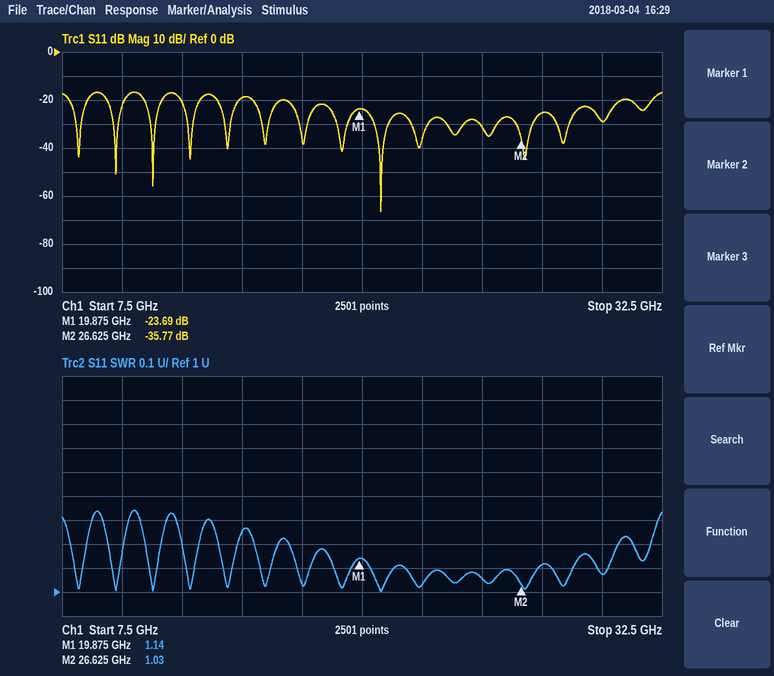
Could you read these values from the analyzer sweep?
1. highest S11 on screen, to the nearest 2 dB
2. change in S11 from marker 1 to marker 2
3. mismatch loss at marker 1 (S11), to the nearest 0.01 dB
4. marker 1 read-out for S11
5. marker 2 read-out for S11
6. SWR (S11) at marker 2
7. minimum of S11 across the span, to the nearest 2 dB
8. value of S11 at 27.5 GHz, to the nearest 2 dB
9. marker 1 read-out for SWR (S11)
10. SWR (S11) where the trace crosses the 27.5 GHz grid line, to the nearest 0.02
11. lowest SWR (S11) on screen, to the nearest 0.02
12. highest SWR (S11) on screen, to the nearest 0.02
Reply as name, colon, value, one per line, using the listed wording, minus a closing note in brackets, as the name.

highest S11 on screen, to the nearest 2 dB: -16 dB
change in S11 from marker 1 to marker 2: -12.08 dB
mismatch loss at marker 1 (S11), to the nearest 0.01 dB: 0.02 dB
marker 1 read-out for S11: -23.69 dB
marker 2 read-out for S11: -35.77 dB
SWR (S11) at marker 2: 1.03
minimum of S11 across the span, to the nearest 2 dB: -66 dB
value of S11 at 27.5 GHz, to the nearest 2 dB: -26 dB
marker 1 read-out for SWR: 1.14
SWR (S11) where the trace crosses the 27.5 GHz grid line, to the nearest 0.02: 1.12
lowest SWR (S11) on screen, to the nearest 0.02: 1.00
highest SWR (S11) on screen, to the nearest 0.02: 1.34
